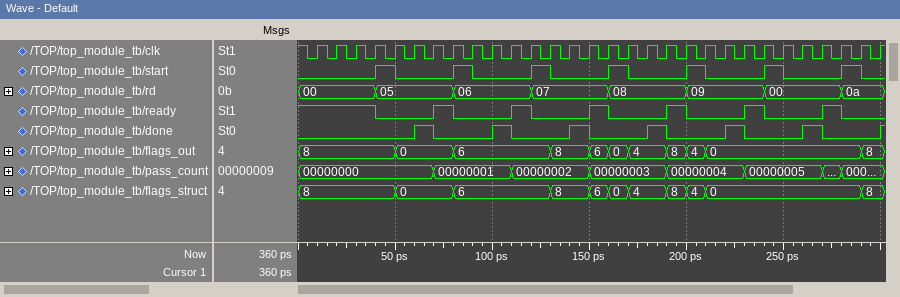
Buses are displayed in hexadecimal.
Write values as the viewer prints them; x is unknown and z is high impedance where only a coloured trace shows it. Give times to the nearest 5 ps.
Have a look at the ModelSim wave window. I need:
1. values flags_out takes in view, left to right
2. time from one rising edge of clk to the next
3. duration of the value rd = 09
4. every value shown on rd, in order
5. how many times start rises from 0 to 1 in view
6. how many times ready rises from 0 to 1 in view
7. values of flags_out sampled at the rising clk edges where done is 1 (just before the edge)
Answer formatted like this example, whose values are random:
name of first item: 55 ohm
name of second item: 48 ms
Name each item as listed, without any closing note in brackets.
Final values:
values flags_out takes in view, left to right: 8, 0, 6, 8, 6, 0, 4, 8, 4, 0, 8
time from one rising edge of clk to the next: 10 ps
duration of the value rd = 09: 40 ps
every value shown on rd, in order: 00, 05, 06, 07, 08, 09, 00, 0a
how many times start rises from 0 to 1 in view: 7
how many times ready rises from 0 to 1 in view: 6
values of flags_out sampled at the rising clk edges where done is 1: 0, 6, 8, 4, 0, 0
